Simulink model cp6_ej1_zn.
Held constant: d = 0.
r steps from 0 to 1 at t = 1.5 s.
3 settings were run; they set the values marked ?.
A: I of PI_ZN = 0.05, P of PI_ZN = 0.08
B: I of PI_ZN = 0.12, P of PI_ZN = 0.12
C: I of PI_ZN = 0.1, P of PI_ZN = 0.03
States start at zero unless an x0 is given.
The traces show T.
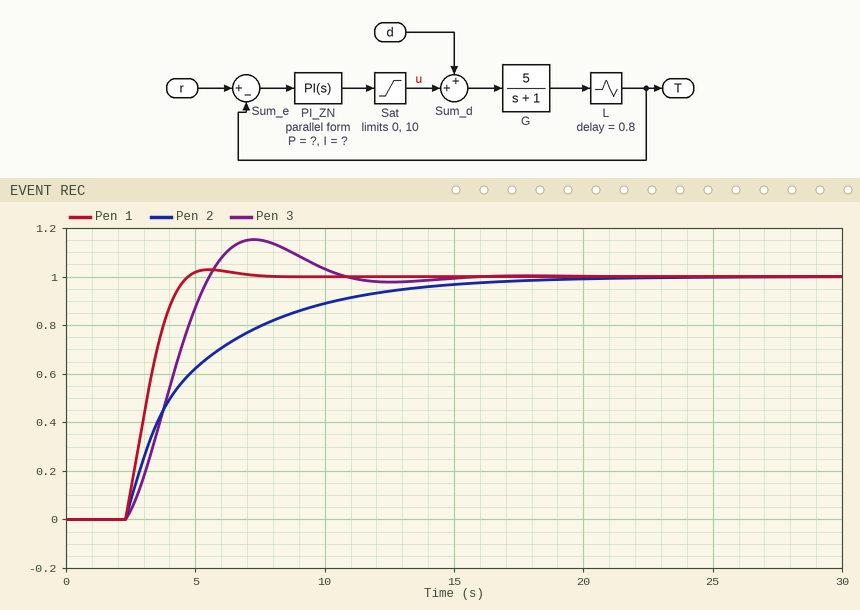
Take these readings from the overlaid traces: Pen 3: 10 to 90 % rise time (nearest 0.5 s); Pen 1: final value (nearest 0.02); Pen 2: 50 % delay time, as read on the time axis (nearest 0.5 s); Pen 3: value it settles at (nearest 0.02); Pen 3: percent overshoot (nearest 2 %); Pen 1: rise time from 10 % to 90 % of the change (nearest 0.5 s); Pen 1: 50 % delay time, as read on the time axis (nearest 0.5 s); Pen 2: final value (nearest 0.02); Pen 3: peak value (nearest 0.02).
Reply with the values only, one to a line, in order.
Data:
2.5 s
1.00
4.0 s
1.00
16 %
1.5 s
3.0 s
1.00
1.16
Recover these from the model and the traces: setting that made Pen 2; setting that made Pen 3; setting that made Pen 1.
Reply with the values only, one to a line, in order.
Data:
A
C
B
